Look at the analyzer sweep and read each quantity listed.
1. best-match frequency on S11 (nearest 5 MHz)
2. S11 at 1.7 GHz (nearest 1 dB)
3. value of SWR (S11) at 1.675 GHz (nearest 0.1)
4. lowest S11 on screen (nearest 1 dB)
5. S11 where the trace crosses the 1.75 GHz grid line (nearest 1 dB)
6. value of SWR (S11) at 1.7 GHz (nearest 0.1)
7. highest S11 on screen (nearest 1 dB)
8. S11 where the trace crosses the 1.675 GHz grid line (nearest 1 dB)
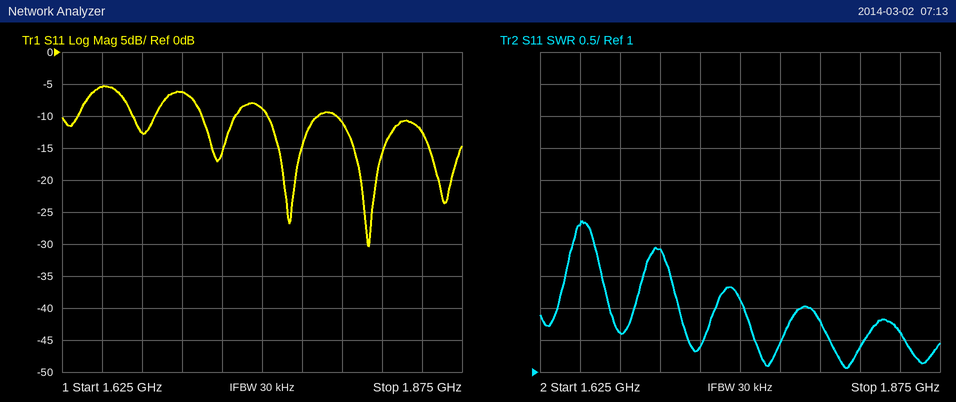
1.815 GHz
-6 dB
1.6
-30 dB
-9 dB
2.9
-5 dB
-13 dB
